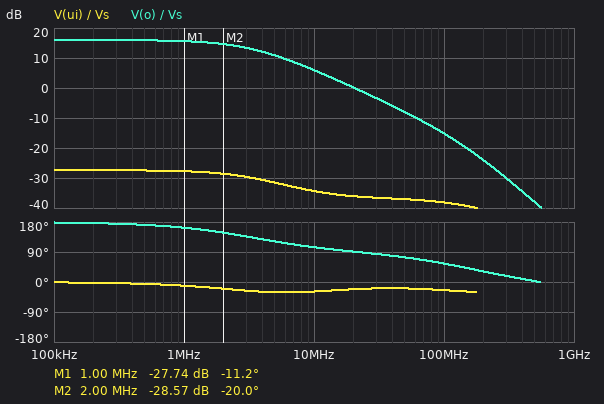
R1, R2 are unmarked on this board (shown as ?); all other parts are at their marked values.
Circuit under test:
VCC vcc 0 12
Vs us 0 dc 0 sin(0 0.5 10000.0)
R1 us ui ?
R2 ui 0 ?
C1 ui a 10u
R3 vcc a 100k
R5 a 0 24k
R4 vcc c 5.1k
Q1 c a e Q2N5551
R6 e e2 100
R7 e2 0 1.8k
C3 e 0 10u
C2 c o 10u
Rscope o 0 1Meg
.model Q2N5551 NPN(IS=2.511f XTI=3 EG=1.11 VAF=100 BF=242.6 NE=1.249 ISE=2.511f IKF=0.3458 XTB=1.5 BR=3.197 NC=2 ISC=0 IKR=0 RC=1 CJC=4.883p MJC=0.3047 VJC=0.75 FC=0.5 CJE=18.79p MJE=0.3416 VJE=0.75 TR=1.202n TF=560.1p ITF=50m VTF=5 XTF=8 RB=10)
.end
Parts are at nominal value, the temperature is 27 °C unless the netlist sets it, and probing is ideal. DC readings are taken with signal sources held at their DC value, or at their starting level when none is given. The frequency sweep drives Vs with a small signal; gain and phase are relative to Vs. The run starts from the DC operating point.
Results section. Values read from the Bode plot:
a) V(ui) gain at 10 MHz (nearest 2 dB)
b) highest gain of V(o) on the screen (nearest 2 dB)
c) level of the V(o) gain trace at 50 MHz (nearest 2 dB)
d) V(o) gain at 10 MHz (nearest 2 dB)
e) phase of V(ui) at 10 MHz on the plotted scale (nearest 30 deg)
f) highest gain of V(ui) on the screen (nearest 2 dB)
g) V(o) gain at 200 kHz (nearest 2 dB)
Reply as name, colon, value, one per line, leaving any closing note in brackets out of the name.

V(ui) gain at 10 MHz: -34 dB
highest gain of V(o) on the screen: 16 dB
level of the V(o) gain trace at 50 MHz: -8 dB
V(o) gain at 10 MHz: 6 dB
phase of V(ui) at 10 MHz on the plotted scale: -30 deg
highest gain of V(ui) on the screen: -28 dB
V(o) gain at 200 kHz: 16 dB
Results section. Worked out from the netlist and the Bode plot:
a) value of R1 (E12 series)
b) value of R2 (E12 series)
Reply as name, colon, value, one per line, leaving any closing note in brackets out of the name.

value of R1: 1.8 kΩ
value of R2: 82 Ω
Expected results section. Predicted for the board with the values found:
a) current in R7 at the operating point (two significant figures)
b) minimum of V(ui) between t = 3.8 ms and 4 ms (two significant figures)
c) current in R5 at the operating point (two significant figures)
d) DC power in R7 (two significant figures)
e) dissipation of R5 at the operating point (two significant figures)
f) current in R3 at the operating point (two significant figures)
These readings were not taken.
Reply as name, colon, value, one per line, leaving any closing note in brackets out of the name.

current in R7 at the operating point: 790 µA
minimum of V(ui) between t = 3.8 ms and 4 ms: -21 mV
current in R5 at the operating point: 91 µA
DC power in R7: 1.1 mW
dissipation of R5 at the operating point: 200 µW
current in R3 at the operating point: 98 µA
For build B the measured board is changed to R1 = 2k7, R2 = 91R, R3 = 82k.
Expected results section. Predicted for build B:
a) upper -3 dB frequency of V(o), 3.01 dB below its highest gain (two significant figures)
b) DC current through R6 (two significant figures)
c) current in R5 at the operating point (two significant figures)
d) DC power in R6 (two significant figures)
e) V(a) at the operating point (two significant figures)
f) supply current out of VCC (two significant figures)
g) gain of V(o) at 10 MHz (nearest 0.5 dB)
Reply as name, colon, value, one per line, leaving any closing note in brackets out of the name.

upper -3 dB frequency of V(o), 3.01 dB below its highest gain: 2.5 MHz
DC current through R6: 980 µA
current in R5 at the operating point: 110 µA
DC power in R6: 97 µW
V(a) at the operating point: 2.6 V
supply current out of VCC: 1.1 mA
gain of V(o) at 10 MHz: 3.0 dB
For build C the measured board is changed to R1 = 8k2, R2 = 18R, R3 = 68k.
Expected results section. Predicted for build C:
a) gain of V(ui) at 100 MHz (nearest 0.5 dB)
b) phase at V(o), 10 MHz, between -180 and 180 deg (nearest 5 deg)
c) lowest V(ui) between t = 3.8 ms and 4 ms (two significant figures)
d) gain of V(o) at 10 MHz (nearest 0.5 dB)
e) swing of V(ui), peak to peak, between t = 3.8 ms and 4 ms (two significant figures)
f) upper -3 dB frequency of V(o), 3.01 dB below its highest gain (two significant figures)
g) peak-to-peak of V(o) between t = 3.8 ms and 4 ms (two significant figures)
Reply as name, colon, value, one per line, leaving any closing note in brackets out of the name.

gain of V(ui) at 100 MHz: -57.5 dB
phase at V(o), 10 MHz, between -180 and 180 deg: 115 deg
lowest V(ui) between t = 3.8 ms and 4 ms: -1.1 mV
gain of V(o) at 10 MHz: -14.0 dB
swing of V(ui), peak to peak, between t = 3.8 ms and 4 ms: 2.2 mV
upper -3 dB frequency of V(o), 3.01 dB below its highest gain: 4.8 MHz
peak-to-peak of V(o) between t = 3.8 ms and 4 ms: 470 mV
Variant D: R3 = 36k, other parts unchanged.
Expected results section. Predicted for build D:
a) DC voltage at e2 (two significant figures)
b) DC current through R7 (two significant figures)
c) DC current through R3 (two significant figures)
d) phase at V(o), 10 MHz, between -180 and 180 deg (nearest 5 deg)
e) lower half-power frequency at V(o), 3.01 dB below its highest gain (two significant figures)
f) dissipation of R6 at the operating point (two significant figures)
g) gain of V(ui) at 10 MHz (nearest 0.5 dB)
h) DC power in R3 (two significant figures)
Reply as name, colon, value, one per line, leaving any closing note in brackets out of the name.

DC voltage at e2: 3.1 V
DC current through R7: 1.7 mA
DC current through R3: 220 µA
phase at V(o), 10 MHz, between -180 and 180 deg: 150 deg
lower half-power frequency at V(o), 3.01 dB below its highest gain: 230 Hz
dissipation of R6 at the operating point: 300 µW
gain of V(ui) at 10 MHz: -34.5 dB
DC power in R3: 1.8 mW
